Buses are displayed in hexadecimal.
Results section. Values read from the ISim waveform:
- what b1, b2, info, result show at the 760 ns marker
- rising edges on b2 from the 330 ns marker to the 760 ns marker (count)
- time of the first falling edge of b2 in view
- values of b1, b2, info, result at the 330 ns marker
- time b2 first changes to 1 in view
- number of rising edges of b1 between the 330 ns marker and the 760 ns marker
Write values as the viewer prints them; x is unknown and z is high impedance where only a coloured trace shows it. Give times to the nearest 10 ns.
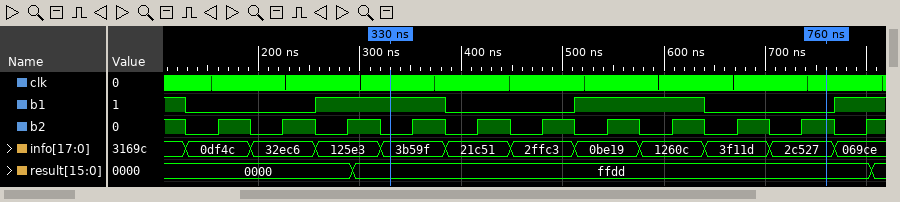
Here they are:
b1=0, b2=1, info=2c527, result=ffdd
7
130 ns
b1=1, b2=0, info=3b59f, result=ffdd
160 ns
1
